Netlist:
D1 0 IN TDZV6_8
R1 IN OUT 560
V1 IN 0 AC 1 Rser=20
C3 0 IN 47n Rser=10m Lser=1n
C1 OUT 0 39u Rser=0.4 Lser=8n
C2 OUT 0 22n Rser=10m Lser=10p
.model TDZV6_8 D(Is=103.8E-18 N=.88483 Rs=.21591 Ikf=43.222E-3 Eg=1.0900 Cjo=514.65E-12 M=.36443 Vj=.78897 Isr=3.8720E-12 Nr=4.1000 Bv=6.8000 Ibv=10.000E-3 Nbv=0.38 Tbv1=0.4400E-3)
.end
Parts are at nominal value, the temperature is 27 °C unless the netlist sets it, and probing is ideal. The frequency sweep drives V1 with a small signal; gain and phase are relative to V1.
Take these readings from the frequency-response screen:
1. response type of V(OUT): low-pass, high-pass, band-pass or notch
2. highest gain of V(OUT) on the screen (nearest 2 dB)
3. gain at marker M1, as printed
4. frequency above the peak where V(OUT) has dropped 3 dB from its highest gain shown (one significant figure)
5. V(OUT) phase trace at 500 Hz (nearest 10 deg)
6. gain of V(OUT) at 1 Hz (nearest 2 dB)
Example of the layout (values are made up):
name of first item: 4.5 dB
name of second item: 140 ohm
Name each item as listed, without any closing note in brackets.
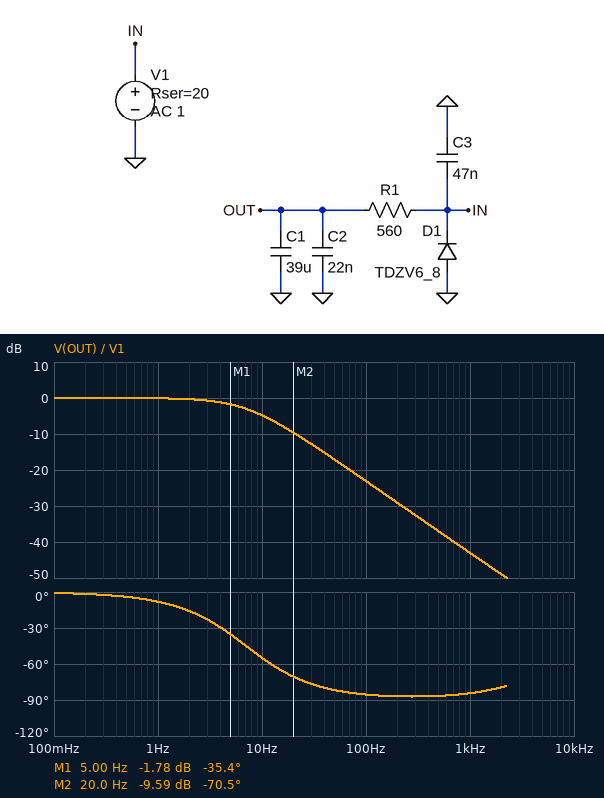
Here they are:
response type of V(OUT): low-pass, high-pass, band-pass or notch: low-pass
highest gain of V(OUT) on the screen: 0 dB
gain at marker M1, as printed: -1.78 dB
frequency above the peak where V(OUT) has dropped 3 dB from its highest gain shown: 7 Hz
V(OUT) phase trace at 500 Hz: -90 deg
gain of V(OUT) at 1 Hz: 0 dB
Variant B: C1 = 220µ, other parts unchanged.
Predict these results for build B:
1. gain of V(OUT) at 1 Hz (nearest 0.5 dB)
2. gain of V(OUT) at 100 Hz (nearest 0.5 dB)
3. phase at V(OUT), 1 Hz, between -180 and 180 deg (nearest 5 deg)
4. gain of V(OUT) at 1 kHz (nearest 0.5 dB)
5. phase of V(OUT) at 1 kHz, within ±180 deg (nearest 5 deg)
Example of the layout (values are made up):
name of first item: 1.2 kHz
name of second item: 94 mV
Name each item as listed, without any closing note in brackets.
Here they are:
gain of V(OUT) at 1 Hz: -2.0 dB
gain of V(OUT) at 100 Hz: -38.0 dB
phase at V(OUT), 1 Hz, between -180 and 180 deg: -40 deg
gain of V(OUT) at 1 kHz: -57.0 dB
phase of V(OUT) at 1 kHz, within ±180 deg: -60 deg
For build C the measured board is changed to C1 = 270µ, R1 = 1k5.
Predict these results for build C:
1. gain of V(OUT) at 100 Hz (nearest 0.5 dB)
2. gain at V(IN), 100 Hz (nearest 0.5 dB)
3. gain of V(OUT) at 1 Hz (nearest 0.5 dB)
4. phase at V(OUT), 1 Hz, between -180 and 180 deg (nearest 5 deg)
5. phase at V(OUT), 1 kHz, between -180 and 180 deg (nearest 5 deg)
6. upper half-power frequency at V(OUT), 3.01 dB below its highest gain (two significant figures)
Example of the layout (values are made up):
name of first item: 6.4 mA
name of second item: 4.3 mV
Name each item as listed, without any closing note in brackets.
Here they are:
gain of V(OUT) at 100 Hz: -48.0 dB
gain at V(IN), 100 Hz: 0 dB
gain of V(OUT) at 1 Hz: -9.0 dB
phase at V(OUT), 1 Hz, between -180 and 180 deg: -70 deg
phase at V(OUT), 1 kHz, between -180 and 180 deg: -55 deg
upper half-power frequency at V(OUT), 3.01 dB below its highest gain: 390 mHz
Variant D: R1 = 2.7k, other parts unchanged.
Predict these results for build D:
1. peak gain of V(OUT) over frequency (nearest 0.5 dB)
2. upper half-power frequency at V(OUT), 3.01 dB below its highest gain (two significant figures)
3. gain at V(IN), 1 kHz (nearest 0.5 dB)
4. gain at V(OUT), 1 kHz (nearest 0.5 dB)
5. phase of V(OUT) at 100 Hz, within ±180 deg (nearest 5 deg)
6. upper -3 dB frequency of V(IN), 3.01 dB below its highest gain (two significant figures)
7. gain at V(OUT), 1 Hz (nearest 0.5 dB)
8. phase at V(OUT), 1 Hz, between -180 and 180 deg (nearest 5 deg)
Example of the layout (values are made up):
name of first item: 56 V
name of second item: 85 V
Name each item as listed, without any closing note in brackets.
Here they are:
peak gain of V(OUT) over frequency: 0 dB
upper half-power frequency at V(OUT), 3.01 dB below its highest gain: 1.5 Hz
gain at V(IN), 1 kHz: 0 dB
gain at V(OUT), 1 kHz: -56.5 dB
phase of V(OUT) at 100 Hz, within ±180 deg: -90 deg
upper -3 dB frequency of V(IN), 3.01 dB below its highest gain: 170 kHz
gain at V(OUT), 1 Hz: -1.5 dB
phase at V(OUT), 1 Hz, between -180 and 180 deg: -35 deg
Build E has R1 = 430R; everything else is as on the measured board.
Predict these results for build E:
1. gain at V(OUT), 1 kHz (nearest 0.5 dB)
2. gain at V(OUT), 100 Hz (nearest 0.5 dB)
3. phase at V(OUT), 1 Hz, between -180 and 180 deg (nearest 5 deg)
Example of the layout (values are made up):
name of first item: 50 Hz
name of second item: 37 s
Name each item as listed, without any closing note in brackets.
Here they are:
gain at V(OUT), 1 kHz: -41.0 dB
gain at V(OUT), 100 Hz: -21.0 dB
phase at V(OUT), 1 Hz, between -180 and 180 deg: -5 deg
